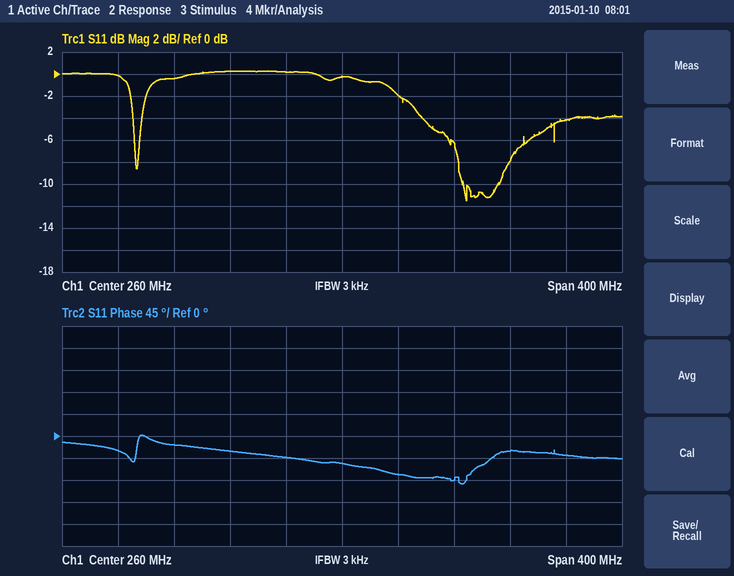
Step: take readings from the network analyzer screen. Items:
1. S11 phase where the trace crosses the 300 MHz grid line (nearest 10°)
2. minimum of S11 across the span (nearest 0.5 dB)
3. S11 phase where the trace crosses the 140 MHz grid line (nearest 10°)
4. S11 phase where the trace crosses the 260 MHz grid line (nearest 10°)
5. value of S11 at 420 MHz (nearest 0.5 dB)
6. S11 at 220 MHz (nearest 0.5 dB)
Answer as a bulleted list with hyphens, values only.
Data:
- -80°
- -11.5 dB
- -20°
- -60°
- -4.0 dB
- 0.0 dB
